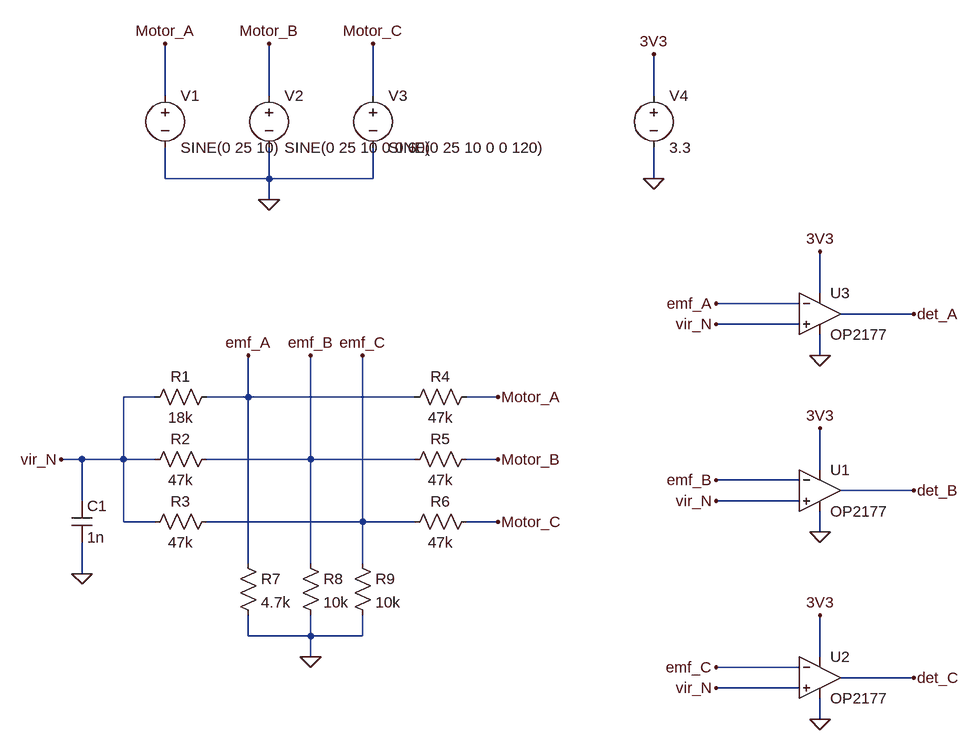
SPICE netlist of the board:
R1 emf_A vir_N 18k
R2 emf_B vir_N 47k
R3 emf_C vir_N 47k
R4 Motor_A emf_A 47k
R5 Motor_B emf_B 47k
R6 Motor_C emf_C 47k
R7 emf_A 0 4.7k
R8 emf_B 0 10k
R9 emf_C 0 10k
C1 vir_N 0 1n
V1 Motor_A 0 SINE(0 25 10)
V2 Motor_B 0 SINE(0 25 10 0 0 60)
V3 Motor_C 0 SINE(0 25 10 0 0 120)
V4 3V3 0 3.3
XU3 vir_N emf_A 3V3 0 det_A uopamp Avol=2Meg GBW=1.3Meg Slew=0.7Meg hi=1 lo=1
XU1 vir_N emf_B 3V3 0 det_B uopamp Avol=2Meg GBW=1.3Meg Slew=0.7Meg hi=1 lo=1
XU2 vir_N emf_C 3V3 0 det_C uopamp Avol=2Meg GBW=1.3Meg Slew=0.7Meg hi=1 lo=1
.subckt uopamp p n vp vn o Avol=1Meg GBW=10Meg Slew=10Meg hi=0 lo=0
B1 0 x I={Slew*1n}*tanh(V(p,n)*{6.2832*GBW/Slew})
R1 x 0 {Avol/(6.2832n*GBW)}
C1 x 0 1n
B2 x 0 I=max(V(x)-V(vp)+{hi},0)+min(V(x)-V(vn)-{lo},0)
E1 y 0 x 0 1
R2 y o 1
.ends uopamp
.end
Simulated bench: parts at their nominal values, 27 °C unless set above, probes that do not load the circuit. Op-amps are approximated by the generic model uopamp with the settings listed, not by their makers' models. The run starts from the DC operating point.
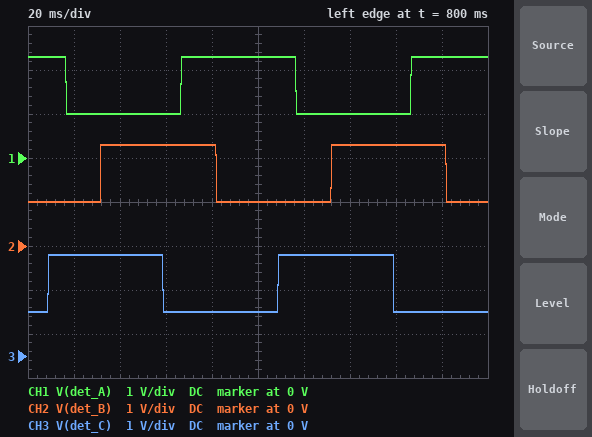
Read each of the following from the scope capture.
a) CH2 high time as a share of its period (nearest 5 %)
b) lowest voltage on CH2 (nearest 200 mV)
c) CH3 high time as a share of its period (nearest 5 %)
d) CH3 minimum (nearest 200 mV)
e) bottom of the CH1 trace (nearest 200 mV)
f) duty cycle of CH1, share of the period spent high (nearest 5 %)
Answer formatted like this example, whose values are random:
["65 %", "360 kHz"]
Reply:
["50 %", "1.0 V", "50 %", "1.0 V", "1.0 V", "50 %"]
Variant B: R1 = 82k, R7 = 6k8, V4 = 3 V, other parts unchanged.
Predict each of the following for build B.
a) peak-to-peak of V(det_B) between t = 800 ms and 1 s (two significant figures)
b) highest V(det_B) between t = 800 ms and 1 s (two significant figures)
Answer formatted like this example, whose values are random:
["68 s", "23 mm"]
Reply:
["1.0 V", "2.0 V"]
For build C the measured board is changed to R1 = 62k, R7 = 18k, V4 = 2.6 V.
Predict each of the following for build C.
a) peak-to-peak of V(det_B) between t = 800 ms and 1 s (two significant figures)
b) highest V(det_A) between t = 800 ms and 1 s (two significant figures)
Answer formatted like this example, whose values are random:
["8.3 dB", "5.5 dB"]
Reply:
["600 mV", "1.6 V"]
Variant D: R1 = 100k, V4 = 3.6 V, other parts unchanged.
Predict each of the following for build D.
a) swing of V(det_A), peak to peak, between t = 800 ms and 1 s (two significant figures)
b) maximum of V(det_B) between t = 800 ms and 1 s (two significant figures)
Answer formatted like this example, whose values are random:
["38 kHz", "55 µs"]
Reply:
["1.6 V", "2.6 V"]
